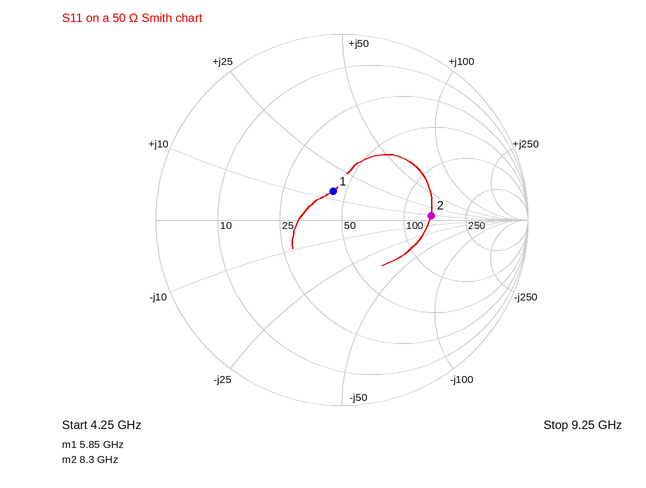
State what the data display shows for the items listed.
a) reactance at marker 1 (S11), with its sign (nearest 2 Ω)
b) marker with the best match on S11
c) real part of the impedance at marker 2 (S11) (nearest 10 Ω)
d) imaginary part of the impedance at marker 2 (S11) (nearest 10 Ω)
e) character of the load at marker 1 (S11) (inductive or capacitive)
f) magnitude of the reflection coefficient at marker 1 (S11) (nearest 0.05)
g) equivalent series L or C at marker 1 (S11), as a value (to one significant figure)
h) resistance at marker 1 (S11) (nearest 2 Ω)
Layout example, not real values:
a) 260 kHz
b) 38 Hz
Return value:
a) +14 Ω
b) marker 1
c) 140 Ω
d) +10 Ω
e) inductive
f) 0.15
g) 400 pH
h) 44 Ω
